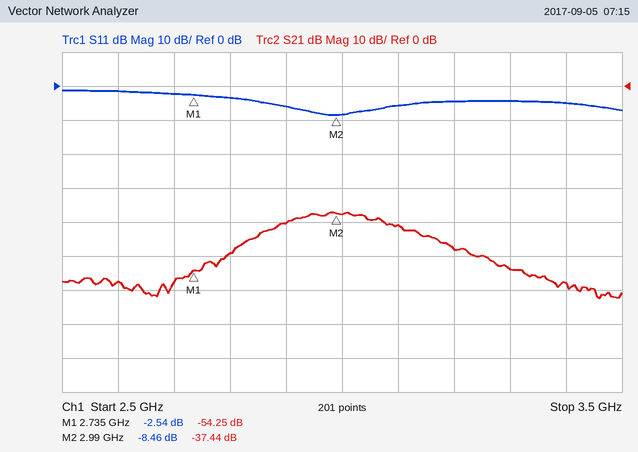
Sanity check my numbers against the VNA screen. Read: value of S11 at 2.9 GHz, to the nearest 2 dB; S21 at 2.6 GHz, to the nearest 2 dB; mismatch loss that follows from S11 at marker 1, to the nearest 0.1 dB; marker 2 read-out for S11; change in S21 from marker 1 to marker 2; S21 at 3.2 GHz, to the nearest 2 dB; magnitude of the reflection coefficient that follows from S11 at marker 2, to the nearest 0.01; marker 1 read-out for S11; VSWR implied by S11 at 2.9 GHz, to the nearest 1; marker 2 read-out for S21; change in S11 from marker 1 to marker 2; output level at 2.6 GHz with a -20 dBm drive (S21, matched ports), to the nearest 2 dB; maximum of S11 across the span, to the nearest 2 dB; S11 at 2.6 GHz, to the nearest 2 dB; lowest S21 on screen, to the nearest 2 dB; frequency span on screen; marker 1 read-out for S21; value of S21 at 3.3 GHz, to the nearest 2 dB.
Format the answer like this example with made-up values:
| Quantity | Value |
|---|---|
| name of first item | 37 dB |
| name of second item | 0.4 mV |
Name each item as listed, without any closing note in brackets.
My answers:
| Quantity | Value |
|---|---|
| value of S11 at 2.9 GHz, to the nearest 2 dB | -6 dB |
| S21 at 2.6 GHz, to the nearest 2 dB | -58 dB |
| mismatch loss that follows from S11 at marker 1, to the nearest 0.1 dB | 3.5 dB |
| marker 2 read-out for S11 | -8.46 dB |
| change in S21 from marker 1 to marker 2 | 16.81 dB |
| S21 at 3.2 GHz, to the nearest 2 dB | -48 dB |
| magnitude of the reflection coefficient that follows from S11 at marker 2, to the nearest 0.01 | 0.38 |
| marker 1 read-out for S11 | -2.54 dB |
| VSWR implied by S11 at 2.9 GHz, to the nearest 1 | 3 |
| marker 2 read-out for S21 | -37.44 dB |
| change in S11 from marker 1 to marker 2 | -5.92 dB |
| output level at 2.6 GHz with a -20 dBm drive (S21, matched ports), to the nearest 2 dB | -78 dBm |
| maximum of S11 across the span, to the nearest 2 dB | -2 dB |
| S11 at 2.6 GHz, to the nearest 2 dB | -2 dB |
| lowest S21 on screen, to the nearest 2 dB | -62 dB |
| frequency span on screen | 1 GHz |
| marker 1 read-out for S21 | -54.25 dB |
| value of S21 at 3.3 GHz, to the nearest 2 dB | -54 dB |
